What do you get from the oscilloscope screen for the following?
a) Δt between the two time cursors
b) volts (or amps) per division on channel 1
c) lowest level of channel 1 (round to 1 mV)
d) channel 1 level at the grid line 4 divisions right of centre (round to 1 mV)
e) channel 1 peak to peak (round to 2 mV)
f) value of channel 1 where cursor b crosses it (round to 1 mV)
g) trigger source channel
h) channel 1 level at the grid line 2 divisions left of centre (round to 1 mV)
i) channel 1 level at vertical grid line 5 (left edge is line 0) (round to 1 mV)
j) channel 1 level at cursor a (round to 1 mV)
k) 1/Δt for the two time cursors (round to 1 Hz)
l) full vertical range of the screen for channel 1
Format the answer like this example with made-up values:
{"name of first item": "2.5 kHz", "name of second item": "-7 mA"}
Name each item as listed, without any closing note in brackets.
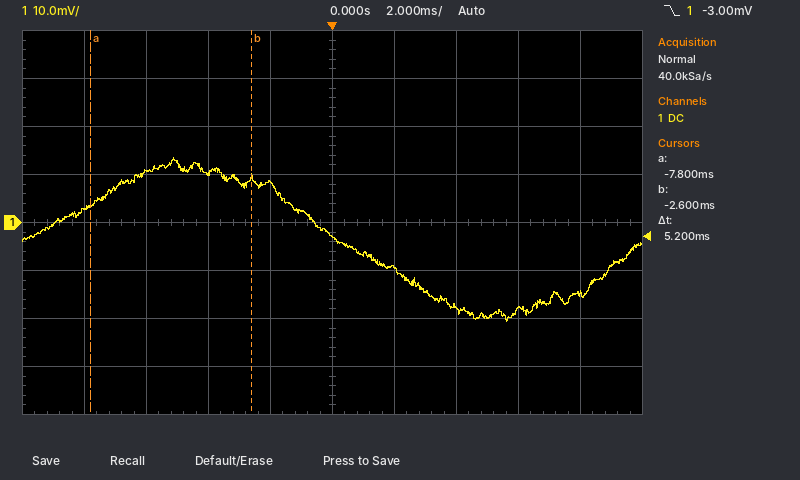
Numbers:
{"Δt between the two time cursors": "5.2 ms", "volts (or amps) per division on channel 1": "10 mV", "lowest level of channel 1": "-21 mV", "channel 1 level at the grid line 4 divisions right of centre": "-15 mV", "channel 1 peak to peak": "34 mV", "value of channel 1 where cursor b crosses it": "9 mV", "trigger source channel": "channel 1", "channel 1 level at the grid line 2 divisions left of centre": "10 mV", "channel 1 level at vertical grid line 5 (left edge is line 0)": "-3 mV", "channel 1 level at cursor a": "3 mV", "1/Δt for the two time cursors": "192 Hz", "full vertical range of the screen for channel 1": "80 mV"}
